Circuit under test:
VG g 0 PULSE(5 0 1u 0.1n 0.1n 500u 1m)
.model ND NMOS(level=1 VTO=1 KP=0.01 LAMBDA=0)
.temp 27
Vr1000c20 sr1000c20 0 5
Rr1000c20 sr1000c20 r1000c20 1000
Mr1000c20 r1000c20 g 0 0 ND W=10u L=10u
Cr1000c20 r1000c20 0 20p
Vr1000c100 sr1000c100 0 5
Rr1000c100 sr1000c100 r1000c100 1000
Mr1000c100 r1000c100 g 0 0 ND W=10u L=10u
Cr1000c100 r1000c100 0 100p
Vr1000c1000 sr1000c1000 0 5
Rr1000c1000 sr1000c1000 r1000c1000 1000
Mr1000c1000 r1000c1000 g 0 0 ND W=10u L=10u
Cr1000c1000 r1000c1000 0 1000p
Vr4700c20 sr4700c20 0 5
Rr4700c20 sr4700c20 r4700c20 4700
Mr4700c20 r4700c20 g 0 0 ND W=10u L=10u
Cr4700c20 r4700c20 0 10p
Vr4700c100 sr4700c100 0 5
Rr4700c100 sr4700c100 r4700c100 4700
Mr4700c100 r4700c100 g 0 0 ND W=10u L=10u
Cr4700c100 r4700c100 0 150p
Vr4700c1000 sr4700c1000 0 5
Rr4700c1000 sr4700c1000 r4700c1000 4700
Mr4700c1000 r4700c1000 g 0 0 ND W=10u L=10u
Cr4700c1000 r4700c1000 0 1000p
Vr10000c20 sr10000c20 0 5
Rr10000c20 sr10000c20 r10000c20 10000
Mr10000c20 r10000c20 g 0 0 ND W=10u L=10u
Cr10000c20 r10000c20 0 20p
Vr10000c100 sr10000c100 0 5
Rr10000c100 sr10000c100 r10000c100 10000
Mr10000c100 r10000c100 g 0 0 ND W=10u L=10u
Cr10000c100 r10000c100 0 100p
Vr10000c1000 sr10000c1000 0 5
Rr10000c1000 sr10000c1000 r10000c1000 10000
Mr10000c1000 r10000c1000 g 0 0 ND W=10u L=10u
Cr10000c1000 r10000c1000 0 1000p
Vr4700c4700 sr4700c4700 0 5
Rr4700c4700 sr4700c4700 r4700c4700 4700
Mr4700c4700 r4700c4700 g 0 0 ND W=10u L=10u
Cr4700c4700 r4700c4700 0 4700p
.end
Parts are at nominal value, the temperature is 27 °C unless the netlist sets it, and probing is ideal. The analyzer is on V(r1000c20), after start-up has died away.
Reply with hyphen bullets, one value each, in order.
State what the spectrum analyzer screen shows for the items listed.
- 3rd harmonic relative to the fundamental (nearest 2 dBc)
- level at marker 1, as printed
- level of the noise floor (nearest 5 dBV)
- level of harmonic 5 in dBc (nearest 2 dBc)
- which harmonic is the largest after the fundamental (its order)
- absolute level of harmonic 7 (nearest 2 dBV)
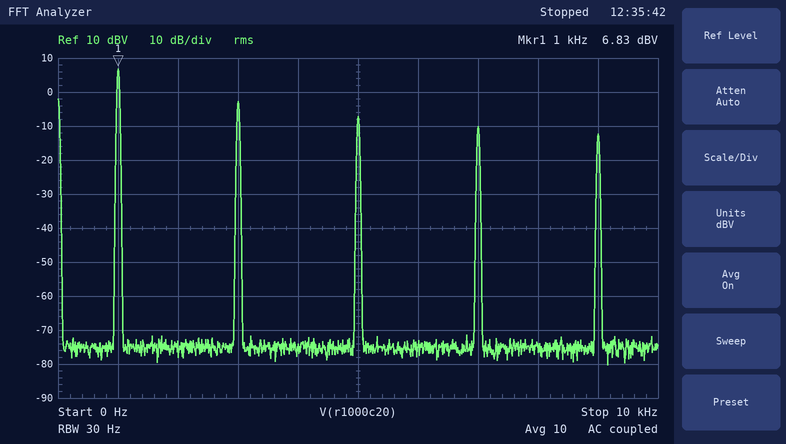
- -10 dBc
- 6.83 dBV
- -75 dBV
- -14 dBc
- 3
- -10 dBV
